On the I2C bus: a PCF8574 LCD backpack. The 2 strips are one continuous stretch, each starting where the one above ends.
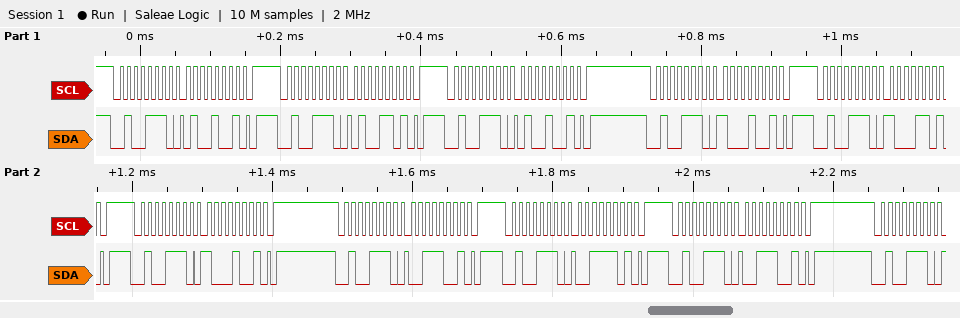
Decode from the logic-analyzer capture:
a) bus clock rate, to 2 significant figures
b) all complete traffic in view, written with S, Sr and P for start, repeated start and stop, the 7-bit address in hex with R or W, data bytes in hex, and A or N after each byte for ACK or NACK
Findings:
100 kHz
S 27W A 49 A P S 27W A 4D A P S 27W A 49 A P S 27W A 89 A P S 27W A 8D A P S 27W A 89 A P S 27W A 39 A P S 27W A 3D A P S 27W A 39 A P S 27W A
